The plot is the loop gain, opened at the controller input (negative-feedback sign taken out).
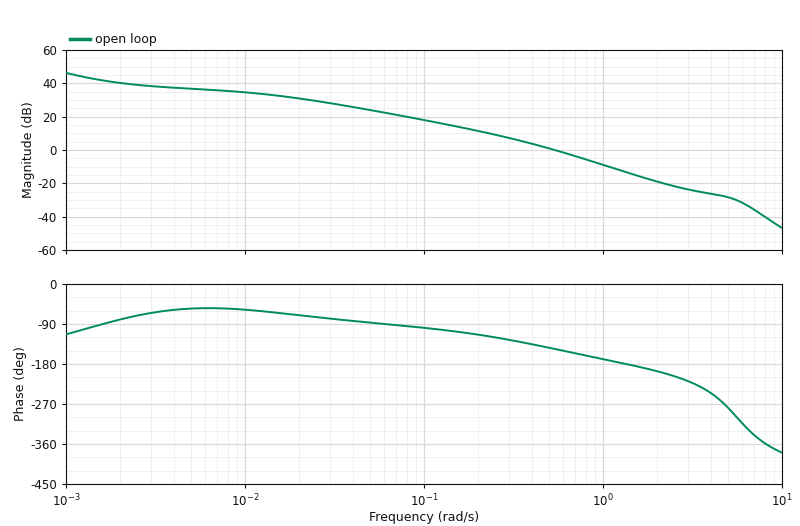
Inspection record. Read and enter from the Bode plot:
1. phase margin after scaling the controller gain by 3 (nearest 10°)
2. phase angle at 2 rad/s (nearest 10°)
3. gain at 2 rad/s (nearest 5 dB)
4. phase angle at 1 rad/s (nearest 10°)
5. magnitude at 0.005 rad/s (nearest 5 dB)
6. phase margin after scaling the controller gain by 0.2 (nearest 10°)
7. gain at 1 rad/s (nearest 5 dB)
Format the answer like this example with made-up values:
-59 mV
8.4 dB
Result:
10°
-200°
-20 dB
-170°
35 dB
70°
-10 dB
